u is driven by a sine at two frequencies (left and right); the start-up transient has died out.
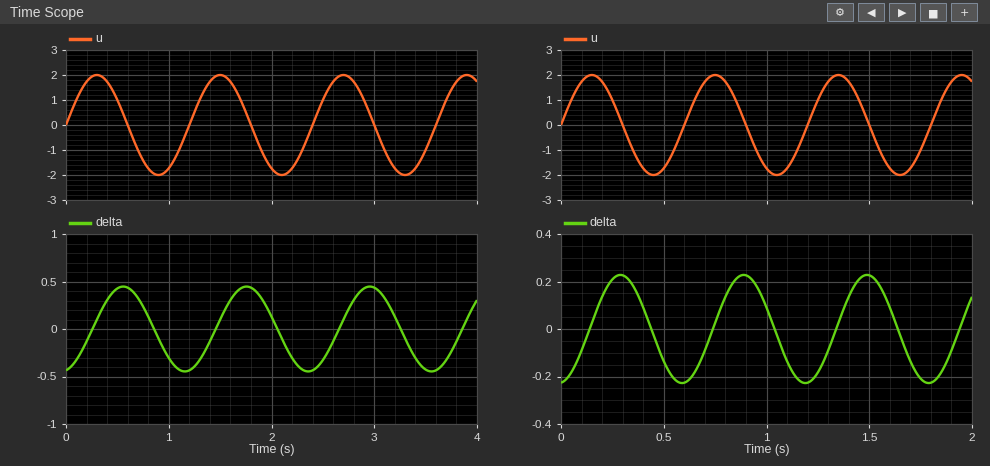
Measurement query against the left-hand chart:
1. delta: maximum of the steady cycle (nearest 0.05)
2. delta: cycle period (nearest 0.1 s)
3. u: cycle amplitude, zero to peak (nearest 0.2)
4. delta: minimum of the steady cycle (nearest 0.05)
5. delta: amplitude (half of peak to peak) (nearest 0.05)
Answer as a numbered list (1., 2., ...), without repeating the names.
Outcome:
1. 0.45
2. 1.2 s
3. 2.0
4. -0.45
5. 0.45
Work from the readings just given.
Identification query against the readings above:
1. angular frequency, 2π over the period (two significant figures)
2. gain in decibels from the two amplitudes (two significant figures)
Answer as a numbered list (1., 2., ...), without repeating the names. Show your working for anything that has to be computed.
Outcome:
1. 2π / 1.2 = 5.2 rad/s
2. 20 log10(0.45 / 2) = -13 dB
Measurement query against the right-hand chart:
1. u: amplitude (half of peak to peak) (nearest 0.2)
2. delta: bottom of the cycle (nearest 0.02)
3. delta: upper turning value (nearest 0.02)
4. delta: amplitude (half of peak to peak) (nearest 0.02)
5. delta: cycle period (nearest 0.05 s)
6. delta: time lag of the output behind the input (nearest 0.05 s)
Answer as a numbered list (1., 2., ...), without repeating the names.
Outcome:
1. 2.0
2. -0.22
3. 0.22
4. 0.22
5. 0.60 s
6. 0.15 s
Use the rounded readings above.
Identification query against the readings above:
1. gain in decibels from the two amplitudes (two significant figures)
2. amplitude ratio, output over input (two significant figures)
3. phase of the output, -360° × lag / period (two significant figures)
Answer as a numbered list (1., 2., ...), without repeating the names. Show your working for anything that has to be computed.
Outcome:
1. 20 log10(0.22 / 2) = -19 dB
2. 0.22 / 2 = 0.11
3. -360 × 0.15 / 0.6 = -90°
